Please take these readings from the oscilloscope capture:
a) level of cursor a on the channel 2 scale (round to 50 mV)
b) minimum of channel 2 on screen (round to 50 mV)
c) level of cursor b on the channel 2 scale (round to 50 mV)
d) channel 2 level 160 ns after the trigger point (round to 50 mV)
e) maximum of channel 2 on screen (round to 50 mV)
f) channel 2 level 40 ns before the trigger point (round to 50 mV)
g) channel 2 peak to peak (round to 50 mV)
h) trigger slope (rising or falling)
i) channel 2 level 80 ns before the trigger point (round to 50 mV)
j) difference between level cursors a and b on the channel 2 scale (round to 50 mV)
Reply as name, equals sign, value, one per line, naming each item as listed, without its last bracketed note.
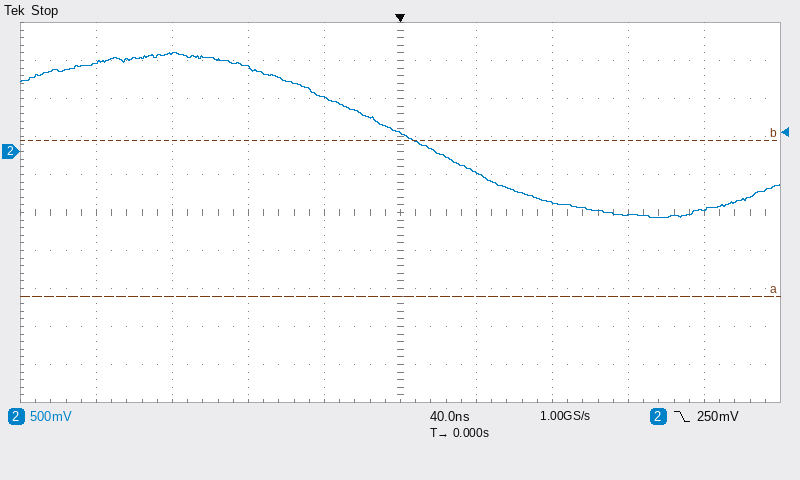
level of cursor a on the channel 2 scale = -1.90 V
minimum of channel 2 on screen = -850 mV
level of cursor b on the channel 2 scale = 150 mV
channel 2 level 160 ns after the trigger point = -750 mV
maximum of channel 2 on screen = 1.30 V
channel 2 level 40 ns before the trigger point = 700 mV
channel 2 peak to peak = 2.15 V
trigger slope = falling
channel 2 level 80 ns before the trigger point = 1.10 V
difference between level cursors a and b on the channel 2 scale = 2.05 V
